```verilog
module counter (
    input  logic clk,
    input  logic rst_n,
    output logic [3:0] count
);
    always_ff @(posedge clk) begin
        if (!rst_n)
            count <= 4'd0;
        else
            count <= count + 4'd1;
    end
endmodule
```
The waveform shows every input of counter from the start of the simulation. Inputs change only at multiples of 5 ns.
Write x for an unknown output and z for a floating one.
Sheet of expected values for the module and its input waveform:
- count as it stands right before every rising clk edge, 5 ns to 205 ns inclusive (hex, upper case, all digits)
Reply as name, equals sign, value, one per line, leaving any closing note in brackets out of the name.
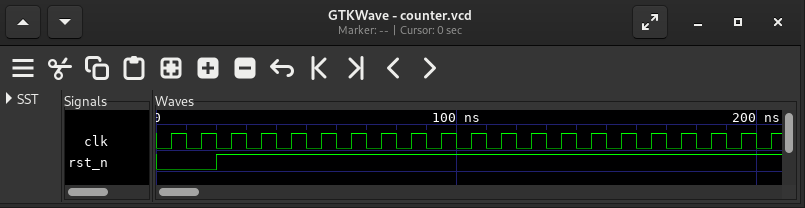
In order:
count as it stands right before every rising clk edge, 5 ns to 205 ns inclusive = x, 0, 0, 1, 2, 3, 4, 5, 6, 7, 8, 9, A, B, C, D, E, F, 0, 1, 2
